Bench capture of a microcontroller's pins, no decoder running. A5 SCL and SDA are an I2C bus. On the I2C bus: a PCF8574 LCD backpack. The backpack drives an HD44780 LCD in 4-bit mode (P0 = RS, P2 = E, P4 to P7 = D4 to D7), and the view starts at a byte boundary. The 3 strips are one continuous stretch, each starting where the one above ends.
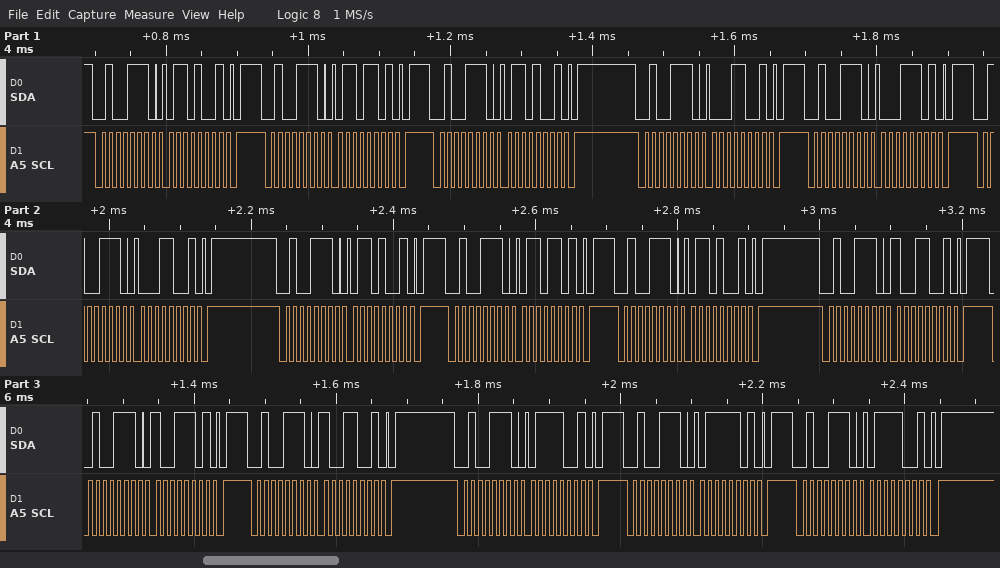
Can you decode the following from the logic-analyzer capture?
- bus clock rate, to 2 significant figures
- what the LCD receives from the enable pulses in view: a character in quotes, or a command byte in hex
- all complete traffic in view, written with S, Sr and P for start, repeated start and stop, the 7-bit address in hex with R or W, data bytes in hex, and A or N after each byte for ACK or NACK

100 kHz
'a' 'i'
S 27W A 69 A P S 27W A 6D A P S 27W A 69 A P S 27W A 19 A P S 27W A 1D A P S 27W A 19 A P S 27W A 69 A P S 27W A 6D A P S 27W A 69 A P S 27W A 99 A P S 27W A 9D A P S 27W A 99 A P S 27W A 79 A P S 27W A 7D A P S 27W A 79 A P
